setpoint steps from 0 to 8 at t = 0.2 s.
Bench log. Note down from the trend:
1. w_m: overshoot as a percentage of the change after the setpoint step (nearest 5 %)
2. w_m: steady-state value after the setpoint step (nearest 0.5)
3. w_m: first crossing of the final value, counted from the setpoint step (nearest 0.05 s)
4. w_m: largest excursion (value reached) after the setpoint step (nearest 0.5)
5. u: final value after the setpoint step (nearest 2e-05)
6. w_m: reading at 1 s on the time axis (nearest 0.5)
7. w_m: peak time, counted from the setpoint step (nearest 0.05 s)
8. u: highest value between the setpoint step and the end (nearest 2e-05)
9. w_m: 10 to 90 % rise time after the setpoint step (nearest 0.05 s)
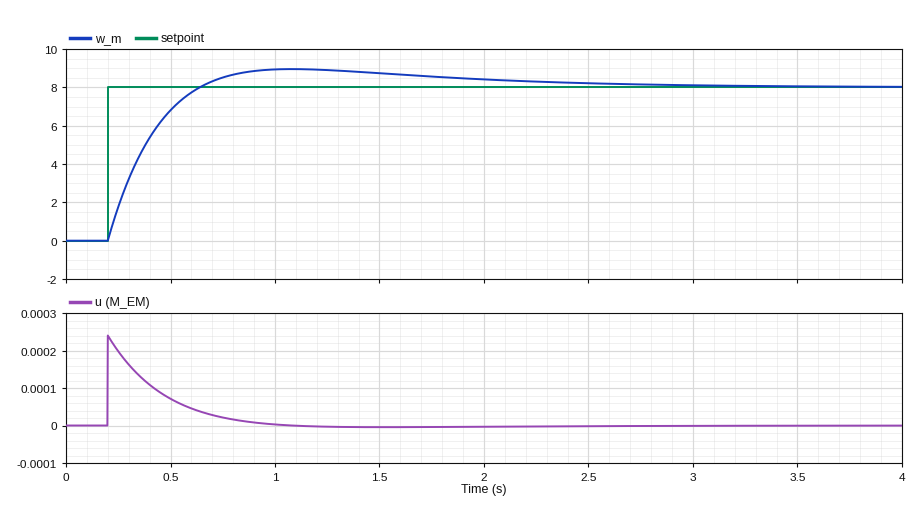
10 %
8.0
0.45 s
9.0
0.00000
9.0
0.90 s
0.00024
0.30 s
